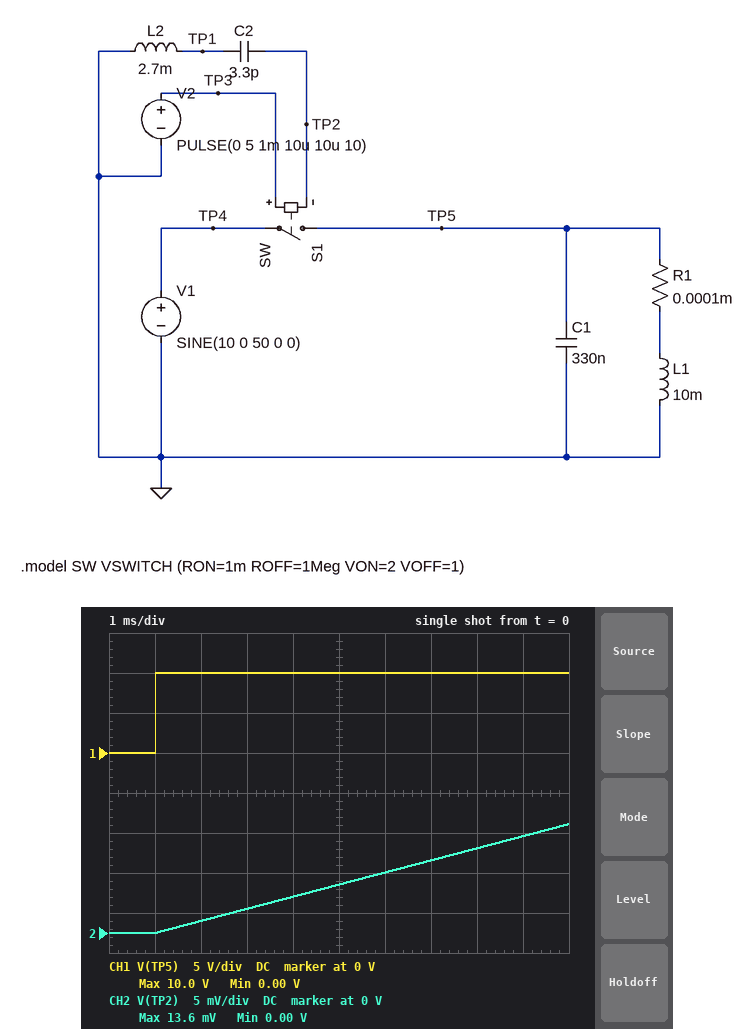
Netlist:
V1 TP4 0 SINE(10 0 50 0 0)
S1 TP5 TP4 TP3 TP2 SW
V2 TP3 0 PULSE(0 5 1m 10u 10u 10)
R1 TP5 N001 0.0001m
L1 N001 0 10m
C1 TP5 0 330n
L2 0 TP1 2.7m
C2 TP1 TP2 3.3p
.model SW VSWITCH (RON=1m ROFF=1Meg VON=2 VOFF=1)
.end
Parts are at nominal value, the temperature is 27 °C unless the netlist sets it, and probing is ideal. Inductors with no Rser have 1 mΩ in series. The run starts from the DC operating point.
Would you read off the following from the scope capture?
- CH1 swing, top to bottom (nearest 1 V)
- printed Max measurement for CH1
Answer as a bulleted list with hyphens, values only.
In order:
- 10 V
- 10.0 V
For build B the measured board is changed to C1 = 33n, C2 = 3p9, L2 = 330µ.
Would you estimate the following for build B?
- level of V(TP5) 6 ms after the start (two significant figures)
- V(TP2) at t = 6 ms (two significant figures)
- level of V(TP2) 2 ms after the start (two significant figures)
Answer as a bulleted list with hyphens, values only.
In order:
- 10 V
- 6.4 mV
- 1.3 mV
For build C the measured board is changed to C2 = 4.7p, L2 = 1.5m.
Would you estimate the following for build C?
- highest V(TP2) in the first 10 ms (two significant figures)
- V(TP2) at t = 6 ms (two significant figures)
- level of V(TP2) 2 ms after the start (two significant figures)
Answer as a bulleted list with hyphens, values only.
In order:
- 9.6 mV
- 5.3 mV
- 1.1 mV
